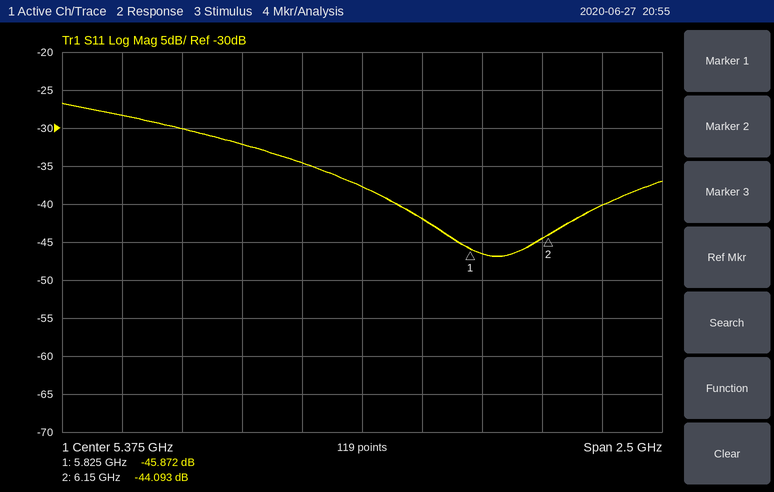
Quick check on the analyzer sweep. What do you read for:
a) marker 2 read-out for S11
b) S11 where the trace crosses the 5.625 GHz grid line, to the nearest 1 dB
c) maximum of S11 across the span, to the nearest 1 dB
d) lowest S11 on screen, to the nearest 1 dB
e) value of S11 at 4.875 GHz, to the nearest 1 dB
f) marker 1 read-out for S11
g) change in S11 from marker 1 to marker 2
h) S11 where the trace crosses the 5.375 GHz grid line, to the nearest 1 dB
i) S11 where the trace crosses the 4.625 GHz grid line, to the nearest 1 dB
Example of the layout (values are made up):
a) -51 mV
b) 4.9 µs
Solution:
a) -44.093 dB
b) -42 dB
c) -27 dB
d) -47 dB
e) -32 dB
f) -45.872 dB
g) 1.779 dB
h) -38 dB
i) -30 dB
